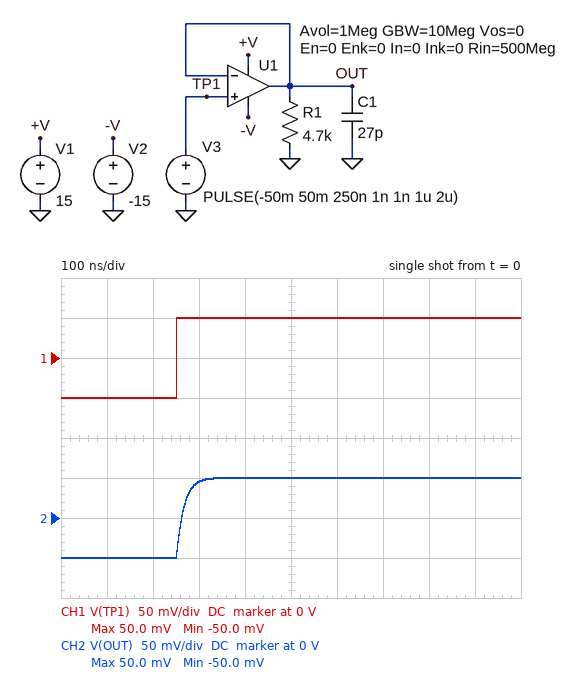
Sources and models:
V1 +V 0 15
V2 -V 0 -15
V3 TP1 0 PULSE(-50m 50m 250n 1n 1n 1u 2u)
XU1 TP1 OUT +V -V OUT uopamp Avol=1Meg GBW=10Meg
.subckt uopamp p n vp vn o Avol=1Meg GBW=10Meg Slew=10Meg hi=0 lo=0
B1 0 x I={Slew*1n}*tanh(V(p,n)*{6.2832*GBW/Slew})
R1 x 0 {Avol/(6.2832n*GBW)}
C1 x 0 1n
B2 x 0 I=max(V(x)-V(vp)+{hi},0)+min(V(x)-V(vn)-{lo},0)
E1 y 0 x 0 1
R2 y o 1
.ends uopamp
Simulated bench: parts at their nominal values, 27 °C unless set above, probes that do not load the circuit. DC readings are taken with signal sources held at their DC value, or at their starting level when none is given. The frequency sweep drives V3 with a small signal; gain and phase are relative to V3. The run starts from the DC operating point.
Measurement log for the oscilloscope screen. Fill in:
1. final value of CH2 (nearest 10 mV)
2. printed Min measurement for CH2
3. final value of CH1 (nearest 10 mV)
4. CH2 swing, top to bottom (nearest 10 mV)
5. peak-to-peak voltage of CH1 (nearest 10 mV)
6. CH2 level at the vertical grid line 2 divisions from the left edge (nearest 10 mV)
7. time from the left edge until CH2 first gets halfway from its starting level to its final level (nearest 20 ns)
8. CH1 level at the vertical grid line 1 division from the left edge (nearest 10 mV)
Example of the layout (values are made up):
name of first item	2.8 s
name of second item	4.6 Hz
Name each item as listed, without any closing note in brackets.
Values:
final value of CH2	50 mV
printed Min measurement for CH2	-50.0 mV
final value of CH1	50 mV
CH2 swing, top to bottom	100 mV
peak-to-peak voltage of CH1	100 mV
CH2 level at the vertical grid line 2 divisions from the left edge	-50 mV
time from the left edge until CH2 first gets halfway from its starting level to its final level	260 ns
CH1 level at the vertical grid line 1 division from the left edge	-50 mV
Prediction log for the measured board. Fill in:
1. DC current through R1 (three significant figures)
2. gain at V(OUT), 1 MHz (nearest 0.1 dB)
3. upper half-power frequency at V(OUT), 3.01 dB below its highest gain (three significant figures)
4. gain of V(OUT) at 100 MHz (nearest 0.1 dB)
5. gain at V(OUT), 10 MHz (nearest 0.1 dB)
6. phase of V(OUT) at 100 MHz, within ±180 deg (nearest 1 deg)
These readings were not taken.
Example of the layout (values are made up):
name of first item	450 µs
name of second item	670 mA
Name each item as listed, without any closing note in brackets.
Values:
DC current through R1	10.6 µA
gain at V(OUT), 1 MHz	0 dB
upper half-power frequency at V(OUT), 3.01 dB below its highest gain	10.0 MHz
gain of V(OUT) at 100 MHz	-20.0 dB
gain at V(OUT), 10 MHz	-3.0 dB
phase of V(OUT) at 100 MHz, within ±180 deg	-85 deg
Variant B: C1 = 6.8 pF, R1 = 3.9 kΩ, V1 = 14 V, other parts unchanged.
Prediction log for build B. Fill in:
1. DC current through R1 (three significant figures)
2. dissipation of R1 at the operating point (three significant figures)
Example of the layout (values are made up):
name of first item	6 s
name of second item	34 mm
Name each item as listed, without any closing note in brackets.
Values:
DC current through R1	12.8 µA
dissipation of R1 at the operating point	641 nW
